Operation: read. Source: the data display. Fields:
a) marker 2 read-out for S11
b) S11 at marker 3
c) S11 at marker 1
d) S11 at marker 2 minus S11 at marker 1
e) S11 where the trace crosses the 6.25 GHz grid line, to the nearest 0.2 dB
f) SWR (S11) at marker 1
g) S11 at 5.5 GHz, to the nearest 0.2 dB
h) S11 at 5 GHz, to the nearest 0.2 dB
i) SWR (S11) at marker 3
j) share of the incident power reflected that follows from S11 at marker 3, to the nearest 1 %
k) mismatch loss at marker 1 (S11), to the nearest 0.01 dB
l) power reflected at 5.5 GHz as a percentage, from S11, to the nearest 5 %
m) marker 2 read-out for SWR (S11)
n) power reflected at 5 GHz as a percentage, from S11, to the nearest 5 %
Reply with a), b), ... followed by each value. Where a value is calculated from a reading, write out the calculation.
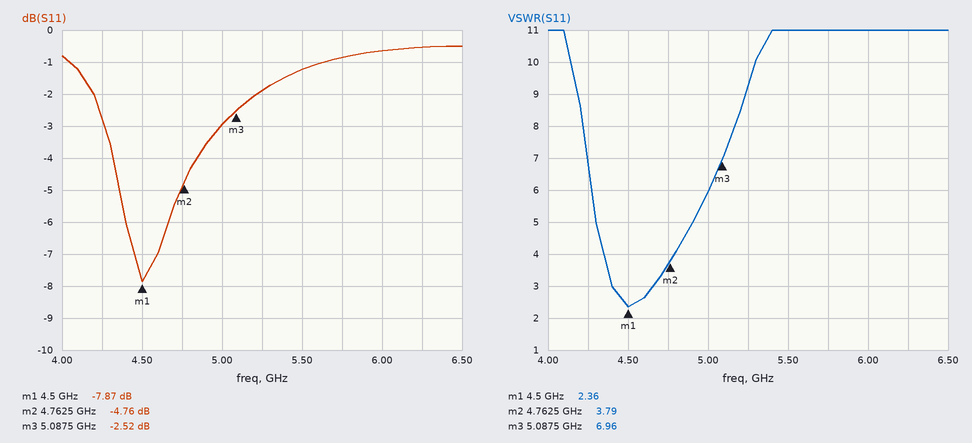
a) -4.76 dB
b) -2.52 dB
c) -7.87 dB
d) -4.76 − (-7.87) = 3.11 dB
e) -0.6 dB
f) 2.36
g) -1.2 dB
h) -3.0 dB
i) 6.96
j) 10^(-2.52/10) ≈ 56 %
k) −10 log10(1 − 10^(-7.87/10)) ≈ 0.77 dB
l) 10^(-1.2/10) ≈ 75.9 %, so 75 % to the nearest 5 %
m) 3.79
n) 10^(-3/10) ≈ 50 %
